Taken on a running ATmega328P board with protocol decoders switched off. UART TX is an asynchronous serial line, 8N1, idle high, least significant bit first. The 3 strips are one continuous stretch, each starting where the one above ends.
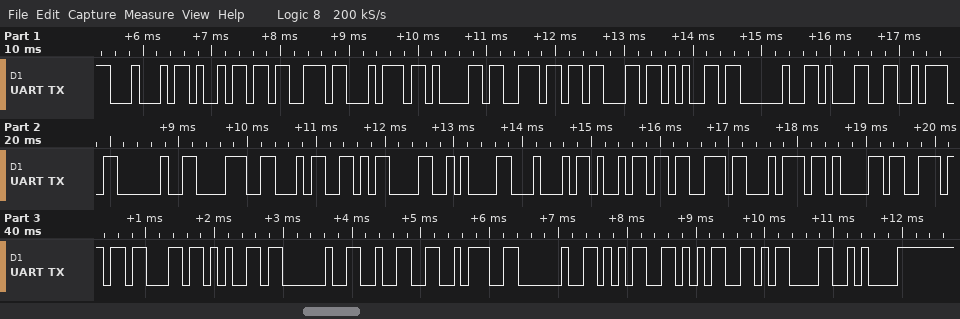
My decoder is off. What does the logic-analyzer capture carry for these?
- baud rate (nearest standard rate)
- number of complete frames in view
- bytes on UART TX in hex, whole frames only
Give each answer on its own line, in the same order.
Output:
9600 baud
32
0x44 0x69 0x73 0x74 0x61 0x6E 0x63 0x65 0x20 0x31 0x3A 0x20 0x38 0x34 0x0D 0x0A 0x44 0x69 0x73 0x74 0x61 0x6E 0x63 0x65 0x20 0x32 0x3A 0x20 0x35 0x35 0x0D 0x0A
